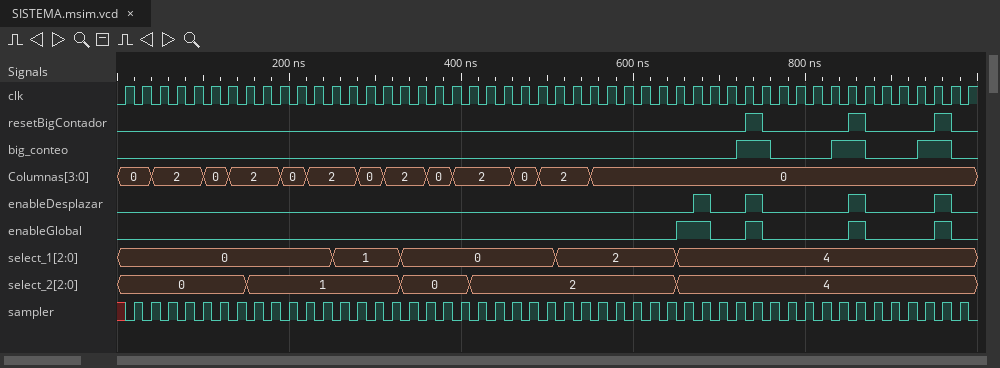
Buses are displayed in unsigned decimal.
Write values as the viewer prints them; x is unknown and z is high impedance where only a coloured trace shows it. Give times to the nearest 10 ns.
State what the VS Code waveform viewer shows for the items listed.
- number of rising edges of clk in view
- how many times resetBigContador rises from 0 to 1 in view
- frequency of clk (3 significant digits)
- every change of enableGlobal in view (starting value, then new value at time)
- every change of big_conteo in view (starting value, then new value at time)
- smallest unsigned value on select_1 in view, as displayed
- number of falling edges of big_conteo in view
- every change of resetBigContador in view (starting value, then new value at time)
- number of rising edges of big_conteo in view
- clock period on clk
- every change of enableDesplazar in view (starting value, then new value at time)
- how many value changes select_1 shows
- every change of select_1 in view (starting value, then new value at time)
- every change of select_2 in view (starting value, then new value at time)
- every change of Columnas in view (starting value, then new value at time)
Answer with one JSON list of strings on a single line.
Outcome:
["50", "3", "50.0 MHz", "0, 1 at 650 ns, 0 at 690 ns, 1 at 730 ns, 0 at 750 ns, 1 at 850 ns, 0 at 870 ns, 1 at 950 ns, 0 at 970 ns", "0, 1 at 720 ns, 0 at 760 ns, 1 at 830 ns, 0 at 870 ns, 1 at 930 ns, 0 at 970 ns", "0", "3", "0, 1 at 730 ns, 0 at 750 ns, 1 at 850 ns, 0 at 870 ns, 1 at 950 ns, 0 at 970 ns", "3", "20 ns", "0, 1 at 670 ns, 0 at 690 ns, 1 at 730 ns, 0 at 750 ns, 1 at 850 ns, 0 at 870 ns, 1 at 950 ns, 0 at 970 ns", "4", "0, 1 at 250 ns, 0 at 330 ns, 2 at 510 ns, 4 at 650 ns", "0, 1 at 150 ns, 0 at 330 ns, 2 at 410 ns, 4 at 650 ns", "0, 2 at 40 ns, 0 at 100 ns, 2 at 130 ns, 0 at 190 ns, 2 at 220 ns, 0 at 280 ns, 2 at 310 ns, 0 at 360 ns, 2 at 390 ns, 0 at 460 ns, 2 at 490 ns, 0 at 550 ns"]
